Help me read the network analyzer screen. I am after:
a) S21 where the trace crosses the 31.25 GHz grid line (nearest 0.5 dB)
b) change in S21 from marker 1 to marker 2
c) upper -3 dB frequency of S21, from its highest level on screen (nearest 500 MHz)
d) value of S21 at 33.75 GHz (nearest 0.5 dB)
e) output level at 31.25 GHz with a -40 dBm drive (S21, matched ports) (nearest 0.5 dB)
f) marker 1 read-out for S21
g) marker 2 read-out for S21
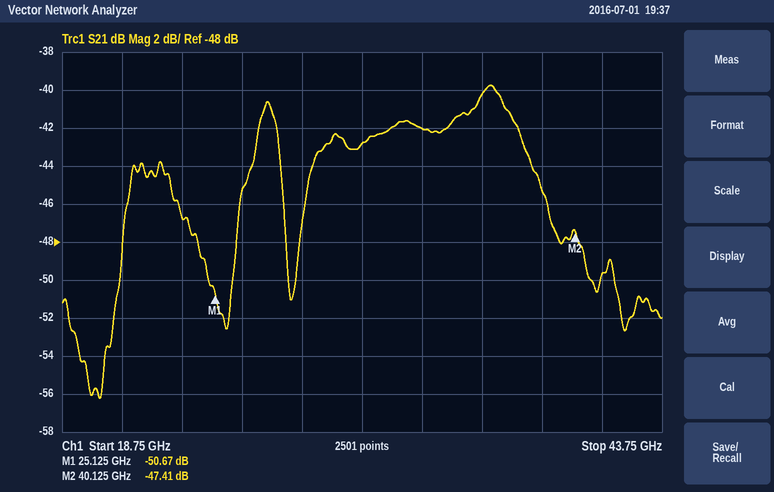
-43.0 dB
3.26 dB
38.0 GHz
-42.0 dB
-83.0 dBm
-50.67 dB
-47.41 dB
